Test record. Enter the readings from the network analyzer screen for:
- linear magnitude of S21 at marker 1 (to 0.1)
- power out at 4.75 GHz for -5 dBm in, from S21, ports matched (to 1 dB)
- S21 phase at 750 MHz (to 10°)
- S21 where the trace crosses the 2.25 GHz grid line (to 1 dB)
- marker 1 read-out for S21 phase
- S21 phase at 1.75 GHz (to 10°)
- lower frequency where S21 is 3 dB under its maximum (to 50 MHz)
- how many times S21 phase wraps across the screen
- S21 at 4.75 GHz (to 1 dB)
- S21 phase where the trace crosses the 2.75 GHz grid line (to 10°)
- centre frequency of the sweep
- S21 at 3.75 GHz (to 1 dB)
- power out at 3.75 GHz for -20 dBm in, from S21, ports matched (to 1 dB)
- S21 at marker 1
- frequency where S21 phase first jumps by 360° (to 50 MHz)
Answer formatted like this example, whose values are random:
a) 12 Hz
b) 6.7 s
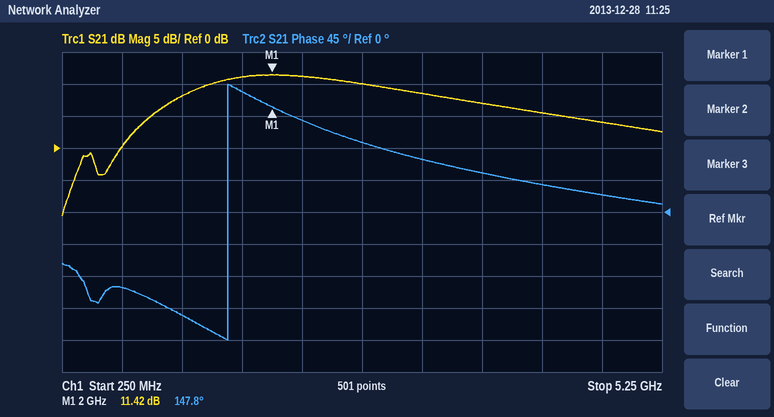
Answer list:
a) 3.7
b) -1 dBm
c) -110°
d) 11 dB
e) 147.8°
f) 170°
g) 1.30 GHz
h) 1
i) 4 dB
j) 100°
k) 2.75 GHz
l) 7 dB
m) -13 dBm
n) 11.42 dB
o) 1.65 GHz
